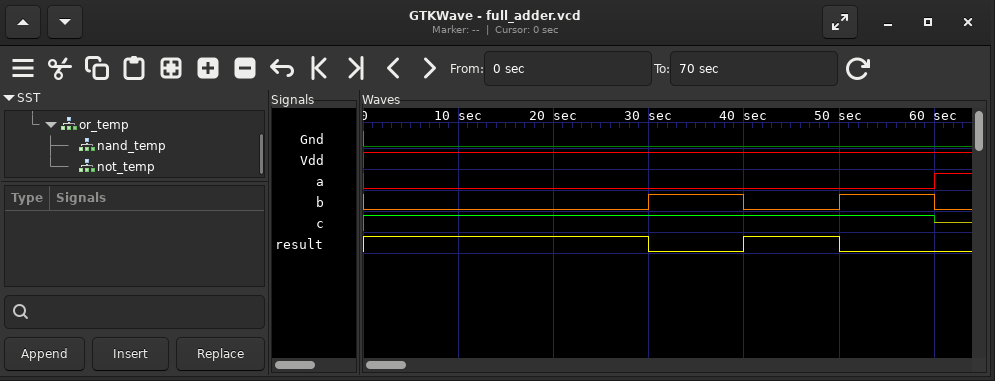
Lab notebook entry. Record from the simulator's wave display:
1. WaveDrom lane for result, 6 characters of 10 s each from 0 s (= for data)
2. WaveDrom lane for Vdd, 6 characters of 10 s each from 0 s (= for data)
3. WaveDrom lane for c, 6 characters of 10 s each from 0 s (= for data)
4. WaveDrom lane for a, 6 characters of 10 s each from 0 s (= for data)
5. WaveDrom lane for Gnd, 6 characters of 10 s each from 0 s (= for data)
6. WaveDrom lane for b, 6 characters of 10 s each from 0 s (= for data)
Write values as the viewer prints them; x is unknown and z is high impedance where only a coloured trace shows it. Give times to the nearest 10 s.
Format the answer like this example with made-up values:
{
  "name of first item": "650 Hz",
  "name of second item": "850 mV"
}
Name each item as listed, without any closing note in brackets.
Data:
{
  "WaveDrom lane for result, 6 characters of 10 s each from 0 s": "{name: 'result', wave: '1..010'}",
  "WaveDrom lane for Vdd, 6 characters of 10 s each from 0 s": "{name: 'Vdd', wave: '1.....'}",
  "WaveDrom lane for c, 6 characters of 10 s each from 0 s": "{name: 'c', wave: '1.....'}",
  "WaveDrom lane for a, 6 characters of 10 s each from 0 s": "{name: 'a', wave: '0.....'}",
  "WaveDrom lane for Gnd, 6 characters of 10 s each from 0 s": "{name: 'Gnd', wave: '0.....'}",
  "WaveDrom lane for b, 6 characters of 10 s each from 0 s": "{name: 'b', wave: '0..101'}"
}
